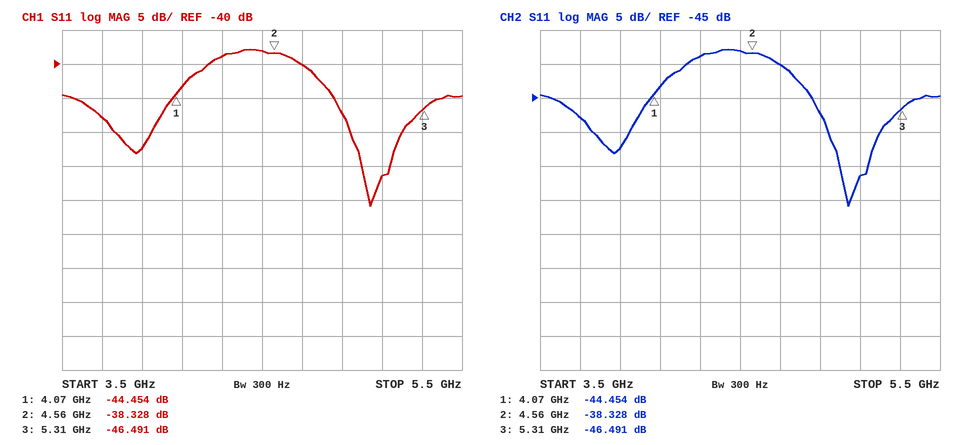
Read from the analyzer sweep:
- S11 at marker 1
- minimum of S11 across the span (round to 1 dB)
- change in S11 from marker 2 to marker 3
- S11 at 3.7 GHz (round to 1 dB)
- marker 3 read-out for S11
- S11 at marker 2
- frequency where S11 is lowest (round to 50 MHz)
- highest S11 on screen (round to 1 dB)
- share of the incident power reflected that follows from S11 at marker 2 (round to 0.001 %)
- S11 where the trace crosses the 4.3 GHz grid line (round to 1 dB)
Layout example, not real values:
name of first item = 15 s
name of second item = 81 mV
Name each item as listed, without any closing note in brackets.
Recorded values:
S11 at marker 1 = -44.454 dB
minimum of S11 across the span = -61 dB
change in S11 from marker 2 to marker 3 = -8.163 dB
S11 at 3.7 GHz = -48 dB
marker 3 read-out for S11 = -46.491 dB
S11 at marker 2 = -38.328 dB
frequency where S11 is lowest = 5.05 GHz
highest S11 on screen = -38 dB
share of the incident power reflected that follows from S11 at marker 2 = 0.015 %
S11 where the trace crosses the 4.3 GHz grid line = -39 dB
